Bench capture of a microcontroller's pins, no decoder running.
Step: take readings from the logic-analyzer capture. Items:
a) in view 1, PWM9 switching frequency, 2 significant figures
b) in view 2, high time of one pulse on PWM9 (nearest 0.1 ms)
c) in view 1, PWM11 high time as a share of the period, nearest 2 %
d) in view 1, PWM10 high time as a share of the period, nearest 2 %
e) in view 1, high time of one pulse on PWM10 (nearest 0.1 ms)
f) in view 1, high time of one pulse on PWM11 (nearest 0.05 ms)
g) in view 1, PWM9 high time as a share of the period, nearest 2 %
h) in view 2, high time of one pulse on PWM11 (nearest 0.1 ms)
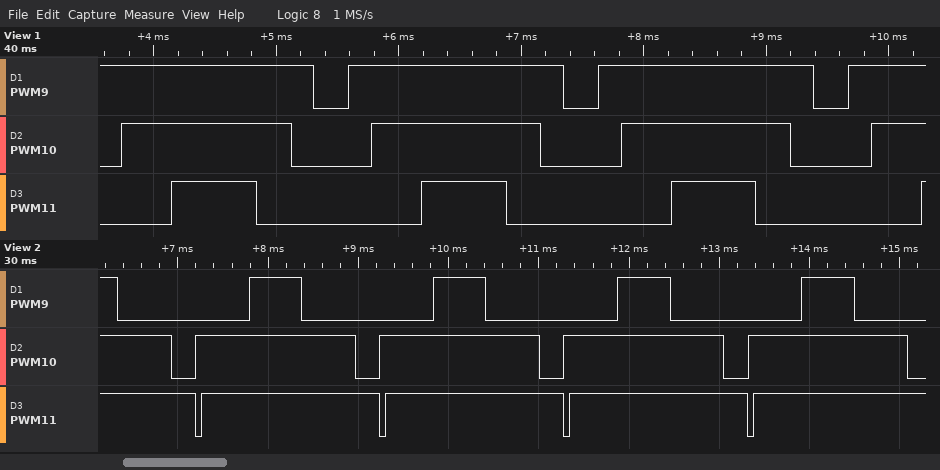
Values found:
490 Hz
0.6 ms
34 %
68 %
1.4 ms
0.70 ms
86 %
2.0 ms
